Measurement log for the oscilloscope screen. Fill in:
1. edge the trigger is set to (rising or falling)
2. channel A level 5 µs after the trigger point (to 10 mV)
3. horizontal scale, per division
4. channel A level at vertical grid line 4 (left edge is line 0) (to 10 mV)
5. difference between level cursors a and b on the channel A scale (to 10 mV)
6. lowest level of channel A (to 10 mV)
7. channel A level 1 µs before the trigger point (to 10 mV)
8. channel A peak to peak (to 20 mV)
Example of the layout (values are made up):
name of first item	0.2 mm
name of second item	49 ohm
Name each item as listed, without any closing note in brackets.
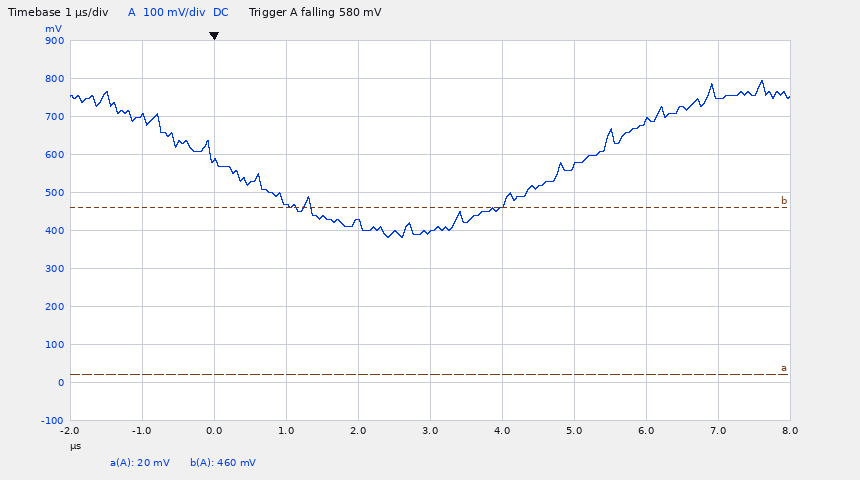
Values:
edge the trigger is set to	falling
channel A level 5 µs after the trigger point	570 mV
horizontal scale, per division	1 µs
channel A level at vertical grid line 4 (left edge is line 0)	420 mV
difference between level cursors a and b on the channel A scale	440 mV
lowest level of channel A	380 mV
channel A level 1 µs before the trigger point	700 mV
channel A peak to peak	420 mV
